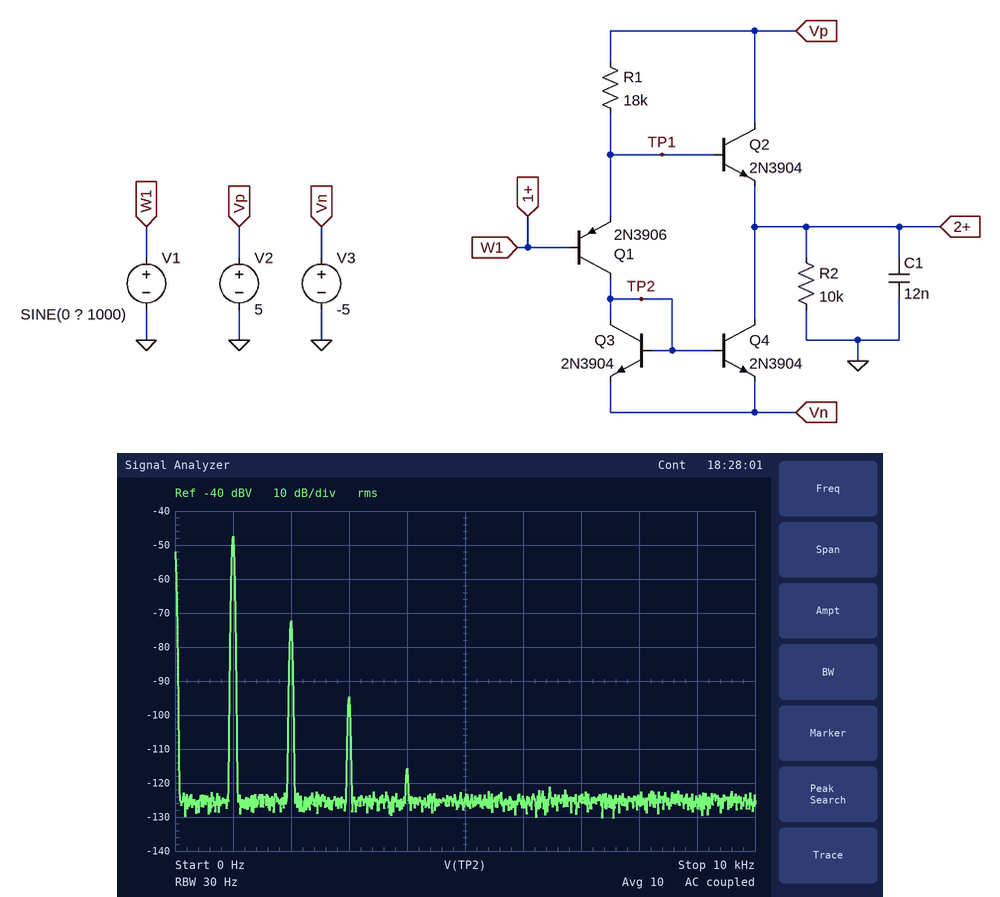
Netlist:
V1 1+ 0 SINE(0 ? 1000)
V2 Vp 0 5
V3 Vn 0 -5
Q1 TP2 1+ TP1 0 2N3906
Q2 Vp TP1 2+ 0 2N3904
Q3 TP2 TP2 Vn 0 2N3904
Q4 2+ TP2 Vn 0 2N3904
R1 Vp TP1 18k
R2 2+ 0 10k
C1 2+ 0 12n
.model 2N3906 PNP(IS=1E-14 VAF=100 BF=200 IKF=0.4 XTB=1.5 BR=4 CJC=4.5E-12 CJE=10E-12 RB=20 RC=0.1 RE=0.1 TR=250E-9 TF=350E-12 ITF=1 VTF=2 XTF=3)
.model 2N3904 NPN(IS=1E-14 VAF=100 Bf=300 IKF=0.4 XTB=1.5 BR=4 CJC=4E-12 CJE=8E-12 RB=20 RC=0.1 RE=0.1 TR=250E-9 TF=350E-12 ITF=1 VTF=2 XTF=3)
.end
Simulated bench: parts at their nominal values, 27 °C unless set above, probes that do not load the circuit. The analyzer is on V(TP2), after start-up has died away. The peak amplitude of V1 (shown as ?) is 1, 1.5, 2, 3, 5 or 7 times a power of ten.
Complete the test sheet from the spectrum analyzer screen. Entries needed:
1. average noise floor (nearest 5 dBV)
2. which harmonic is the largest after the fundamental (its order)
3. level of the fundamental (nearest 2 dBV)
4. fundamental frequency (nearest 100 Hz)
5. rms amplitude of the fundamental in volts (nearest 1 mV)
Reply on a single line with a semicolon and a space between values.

-125 dBV; 2; -48 dBV; 1.0 kHz; 4 mV
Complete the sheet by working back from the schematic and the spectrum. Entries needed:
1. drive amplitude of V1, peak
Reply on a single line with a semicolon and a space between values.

1 V
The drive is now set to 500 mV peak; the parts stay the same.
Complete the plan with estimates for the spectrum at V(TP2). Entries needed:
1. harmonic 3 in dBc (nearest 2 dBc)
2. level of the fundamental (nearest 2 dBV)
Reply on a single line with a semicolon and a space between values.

-60 dBc; -54 dBV
